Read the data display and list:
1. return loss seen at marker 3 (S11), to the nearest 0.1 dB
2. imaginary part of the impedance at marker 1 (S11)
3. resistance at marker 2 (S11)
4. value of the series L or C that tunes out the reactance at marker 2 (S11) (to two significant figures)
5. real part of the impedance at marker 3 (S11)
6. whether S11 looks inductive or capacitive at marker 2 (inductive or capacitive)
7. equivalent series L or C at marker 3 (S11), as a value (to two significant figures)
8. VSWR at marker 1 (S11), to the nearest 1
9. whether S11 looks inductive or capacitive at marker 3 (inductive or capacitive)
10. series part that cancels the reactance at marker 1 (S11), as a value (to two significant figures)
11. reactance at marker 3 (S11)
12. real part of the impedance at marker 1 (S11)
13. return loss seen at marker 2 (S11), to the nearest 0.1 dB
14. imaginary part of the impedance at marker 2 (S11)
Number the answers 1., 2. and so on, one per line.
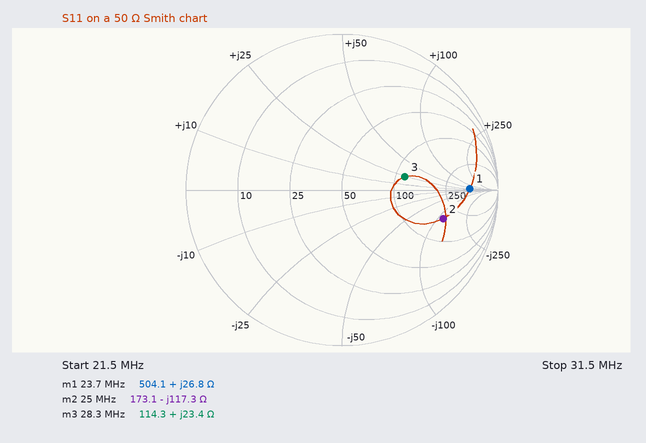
1. 7.7 dB
2. +26.8 Ω
3. 173.1 Ω
4. 750 nH
5. 114.3 Ω
6. capacitive
7. 130 nH
8. 10
9. inductive
10. 250 pF
11. +23.4 Ω
12. 504.1 Ω
13. 3.4 dB
14. -117.3 Ω
